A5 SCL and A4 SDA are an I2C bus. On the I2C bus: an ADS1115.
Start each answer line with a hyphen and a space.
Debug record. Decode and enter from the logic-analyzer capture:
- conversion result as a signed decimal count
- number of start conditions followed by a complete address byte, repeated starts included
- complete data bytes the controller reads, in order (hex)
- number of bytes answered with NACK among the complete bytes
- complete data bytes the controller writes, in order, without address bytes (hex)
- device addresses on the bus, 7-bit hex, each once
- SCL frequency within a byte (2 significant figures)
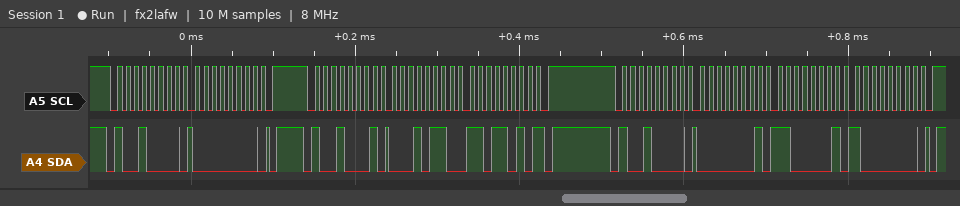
- 5850
- 3
- 16 DA
- 1
- 00 01 C1 80
- 0x48
- 100 kHz
